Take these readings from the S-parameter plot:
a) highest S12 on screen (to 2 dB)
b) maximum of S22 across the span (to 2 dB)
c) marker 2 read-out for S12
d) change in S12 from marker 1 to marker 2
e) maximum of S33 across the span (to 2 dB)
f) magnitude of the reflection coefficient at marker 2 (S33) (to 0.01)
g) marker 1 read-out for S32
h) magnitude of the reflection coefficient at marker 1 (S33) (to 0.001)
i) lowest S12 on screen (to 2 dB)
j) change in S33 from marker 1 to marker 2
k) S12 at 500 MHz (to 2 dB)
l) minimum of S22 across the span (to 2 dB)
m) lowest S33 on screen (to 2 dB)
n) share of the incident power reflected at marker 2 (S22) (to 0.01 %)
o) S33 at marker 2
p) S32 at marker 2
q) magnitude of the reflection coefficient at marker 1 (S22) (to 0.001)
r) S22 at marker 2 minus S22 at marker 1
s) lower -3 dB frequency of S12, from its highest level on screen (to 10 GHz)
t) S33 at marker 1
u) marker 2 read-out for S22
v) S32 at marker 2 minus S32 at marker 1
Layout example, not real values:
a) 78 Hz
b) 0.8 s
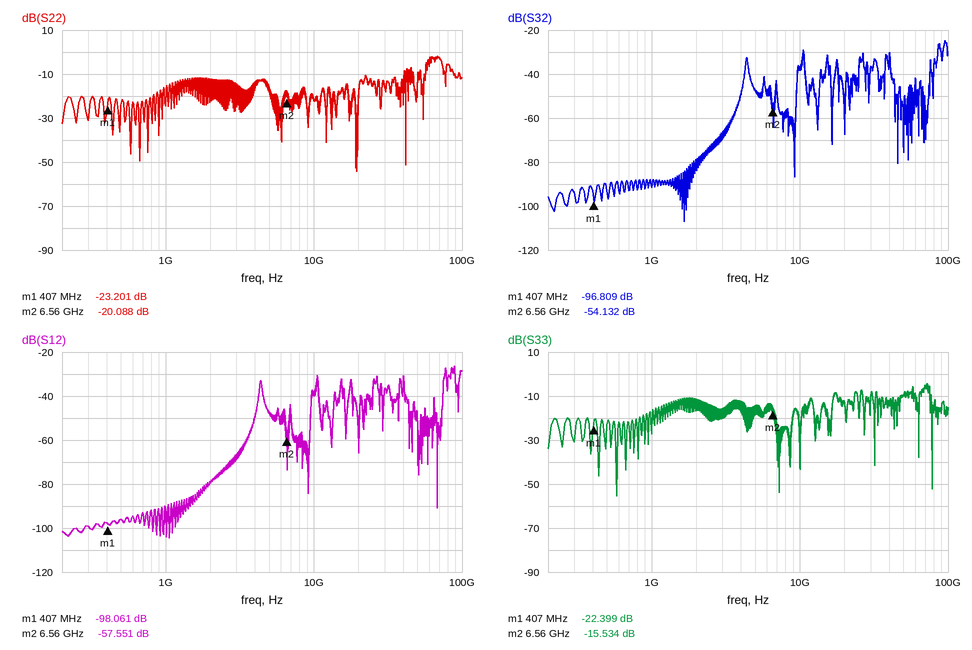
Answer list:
a) -26 dB
b) -2 dB
c) -57.551 dB
d) 40.510 dB
e) -4 dB
f) 0.17
g) -96.809 dB
h) 0.076
i) -104 dB
j) 6.865 dB
k) -96 dB
l) -54 dB
m) -56 dB
n) 0.98 %
o) -15.534 dB
p) -54.132 dB
q) 0.069
r) 3.113 dB
s) 90 GHz
t) -22.399 dB
u) -20.088 dB
v) 42.677 dB
